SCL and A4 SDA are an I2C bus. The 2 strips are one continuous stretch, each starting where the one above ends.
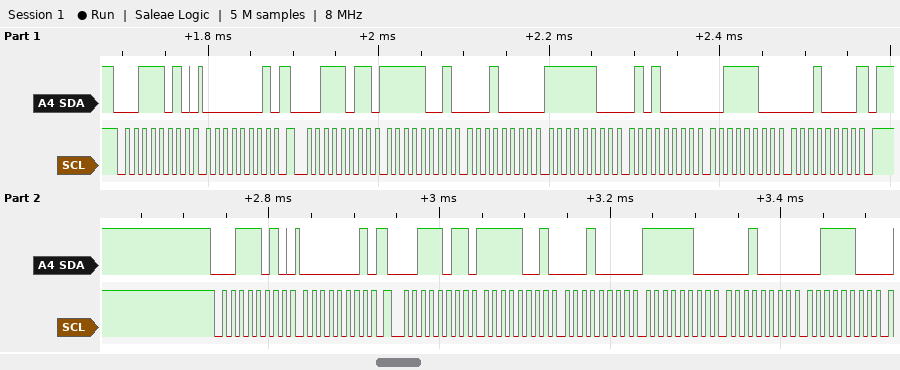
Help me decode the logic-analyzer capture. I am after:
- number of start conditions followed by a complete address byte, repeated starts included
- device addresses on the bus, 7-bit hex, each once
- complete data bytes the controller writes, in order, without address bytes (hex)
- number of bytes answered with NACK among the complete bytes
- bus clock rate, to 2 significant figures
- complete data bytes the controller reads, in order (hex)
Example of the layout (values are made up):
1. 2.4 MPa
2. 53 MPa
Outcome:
1. 4
2. 0x1D
3. 01 01
4. 1
5. 100 kHz
6. F9 10 FC 50 3C 10 F9 10 FC 10 3C
